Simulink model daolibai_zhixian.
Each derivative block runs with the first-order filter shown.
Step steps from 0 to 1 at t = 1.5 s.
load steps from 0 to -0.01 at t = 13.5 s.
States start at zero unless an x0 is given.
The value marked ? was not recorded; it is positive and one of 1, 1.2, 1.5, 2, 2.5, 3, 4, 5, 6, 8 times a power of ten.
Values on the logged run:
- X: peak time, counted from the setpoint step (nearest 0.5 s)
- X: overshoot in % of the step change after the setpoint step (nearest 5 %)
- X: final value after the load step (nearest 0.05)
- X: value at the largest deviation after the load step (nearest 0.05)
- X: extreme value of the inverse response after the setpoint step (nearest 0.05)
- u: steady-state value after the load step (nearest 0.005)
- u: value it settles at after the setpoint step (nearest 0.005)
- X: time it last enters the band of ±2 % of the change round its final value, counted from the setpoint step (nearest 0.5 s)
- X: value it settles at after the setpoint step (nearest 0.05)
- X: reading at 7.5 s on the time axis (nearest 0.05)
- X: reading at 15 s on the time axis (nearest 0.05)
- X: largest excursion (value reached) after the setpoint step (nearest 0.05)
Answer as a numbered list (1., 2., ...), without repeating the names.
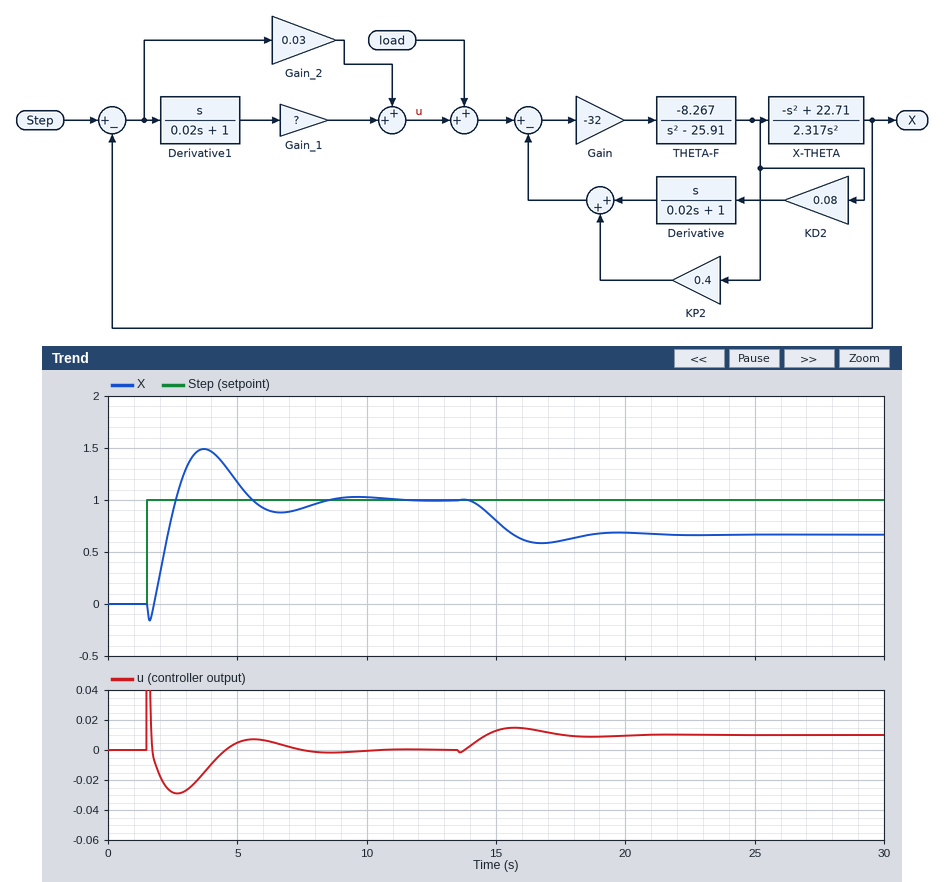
1. 2.0 s
2. 50 %
3. 0.65
4. 0.60
5. -0.15
6. 0.010
7. 0.000
8. 9.0 s
9. 1.00
10. 0.90
11. 0.80
12. 1.50
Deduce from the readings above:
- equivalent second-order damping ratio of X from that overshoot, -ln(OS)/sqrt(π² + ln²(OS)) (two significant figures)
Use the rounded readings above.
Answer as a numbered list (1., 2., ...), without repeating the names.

1. 0.22
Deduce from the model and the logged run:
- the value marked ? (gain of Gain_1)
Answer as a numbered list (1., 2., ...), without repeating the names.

1. 0.03
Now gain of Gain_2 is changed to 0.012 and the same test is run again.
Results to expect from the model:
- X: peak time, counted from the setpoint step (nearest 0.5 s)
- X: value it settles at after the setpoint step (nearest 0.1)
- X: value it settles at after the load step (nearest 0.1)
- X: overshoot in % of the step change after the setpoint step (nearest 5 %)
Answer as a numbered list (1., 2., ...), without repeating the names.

1. 3.0 s
2. 1.0
3. 0.2
4. 25 %
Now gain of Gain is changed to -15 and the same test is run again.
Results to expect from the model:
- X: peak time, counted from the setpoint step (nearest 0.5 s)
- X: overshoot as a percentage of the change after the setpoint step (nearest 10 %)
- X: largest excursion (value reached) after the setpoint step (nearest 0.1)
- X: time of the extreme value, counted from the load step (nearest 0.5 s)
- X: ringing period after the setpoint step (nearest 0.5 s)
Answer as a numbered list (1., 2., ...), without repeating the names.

1. 1.5 s
2. 80 %
3. 1.8
4. 2.5 s
5. 3.5 s
